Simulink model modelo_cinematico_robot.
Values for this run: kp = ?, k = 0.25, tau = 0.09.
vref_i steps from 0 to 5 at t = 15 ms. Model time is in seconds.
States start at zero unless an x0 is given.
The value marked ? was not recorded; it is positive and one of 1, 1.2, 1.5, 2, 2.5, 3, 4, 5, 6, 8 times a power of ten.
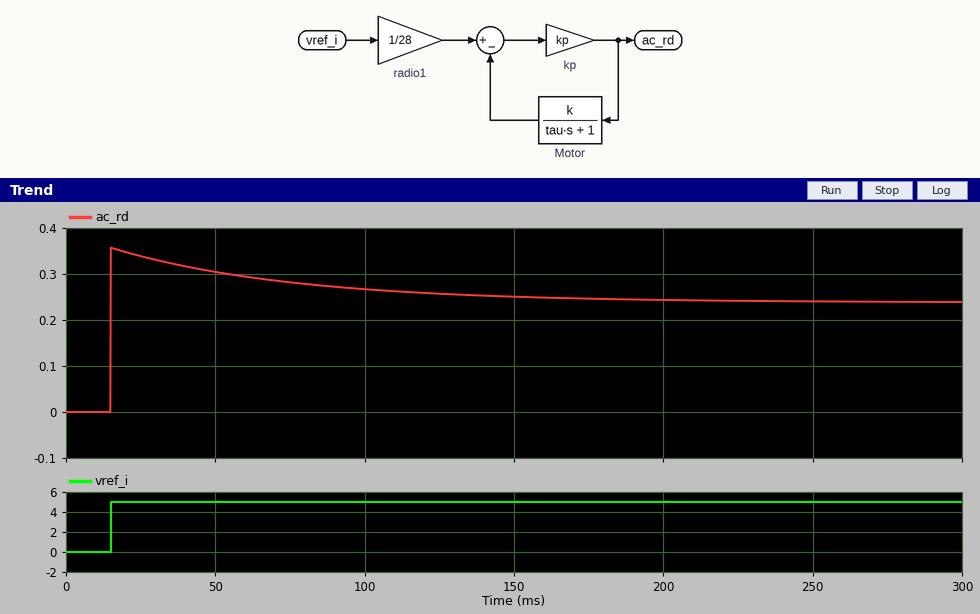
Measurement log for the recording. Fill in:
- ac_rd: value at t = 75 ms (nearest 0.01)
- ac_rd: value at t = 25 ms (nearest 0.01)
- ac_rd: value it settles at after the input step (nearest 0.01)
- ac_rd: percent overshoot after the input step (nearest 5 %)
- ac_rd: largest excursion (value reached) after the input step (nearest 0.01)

0.28
0.34
0.24
50 %
0.36
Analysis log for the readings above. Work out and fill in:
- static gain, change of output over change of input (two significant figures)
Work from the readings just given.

0.048
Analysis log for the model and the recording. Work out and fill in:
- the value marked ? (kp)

2
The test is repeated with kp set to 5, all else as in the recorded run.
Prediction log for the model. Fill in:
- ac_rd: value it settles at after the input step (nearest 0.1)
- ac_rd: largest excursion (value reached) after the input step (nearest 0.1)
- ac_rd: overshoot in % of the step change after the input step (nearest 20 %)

0.4
0.9
120 %
